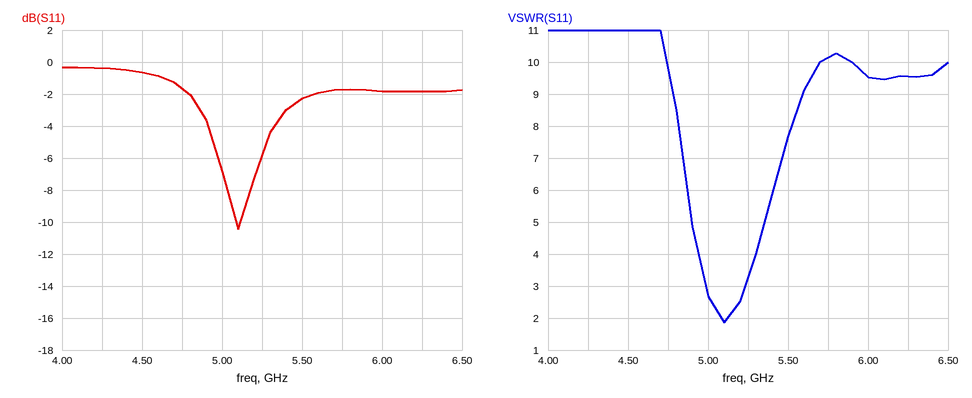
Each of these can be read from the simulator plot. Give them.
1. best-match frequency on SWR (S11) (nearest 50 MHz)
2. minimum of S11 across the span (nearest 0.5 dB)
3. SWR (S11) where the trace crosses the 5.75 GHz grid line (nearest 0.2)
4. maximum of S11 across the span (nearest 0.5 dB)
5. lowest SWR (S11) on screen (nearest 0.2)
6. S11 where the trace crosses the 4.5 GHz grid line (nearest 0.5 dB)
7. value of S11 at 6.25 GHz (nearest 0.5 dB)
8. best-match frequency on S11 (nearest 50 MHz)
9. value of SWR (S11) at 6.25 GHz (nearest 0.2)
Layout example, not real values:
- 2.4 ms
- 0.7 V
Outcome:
- 5.10 GHz
- -10.5 dB
- 10.2
- -0.5 dB
- 1.8
- -0.5 dB
- -2.0 dB
- 5.10 GHz
- 9.6
